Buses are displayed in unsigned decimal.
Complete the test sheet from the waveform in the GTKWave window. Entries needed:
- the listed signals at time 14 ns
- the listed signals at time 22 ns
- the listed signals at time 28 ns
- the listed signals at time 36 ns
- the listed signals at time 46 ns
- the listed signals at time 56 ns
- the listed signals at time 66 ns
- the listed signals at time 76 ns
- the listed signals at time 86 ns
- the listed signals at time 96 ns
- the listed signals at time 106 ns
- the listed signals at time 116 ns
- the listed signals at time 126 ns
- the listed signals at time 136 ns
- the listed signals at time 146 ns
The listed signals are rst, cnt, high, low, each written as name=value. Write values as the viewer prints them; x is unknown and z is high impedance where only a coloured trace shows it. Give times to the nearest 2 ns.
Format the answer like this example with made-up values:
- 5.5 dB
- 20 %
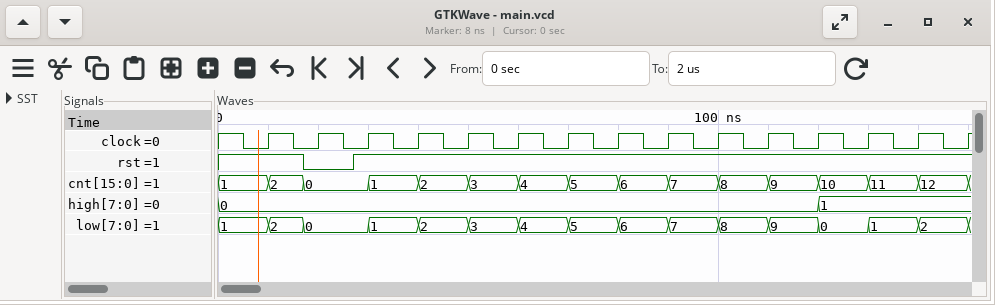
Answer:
- rst=1, cnt=2, high=0, low=2
- rst=0, cnt=0, high=0, low=0
- rst=1, cnt=0, high=0, low=0
- rst=1, cnt=1, high=0, low=1
- rst=1, cnt=2, high=0, low=2
- rst=1, cnt=3, high=0, low=3
- rst=1, cnt=4, high=0, low=4
- rst=1, cnt=5, high=0, low=5
- rst=1, cnt=6, high=0, low=6
- rst=1, cnt=7, high=0, low=7
- rst=1, cnt=8, high=0, low=8
- rst=1, cnt=9, high=0, low=9
- rst=1, cnt=10, high=1, low=0
- rst=1, cnt=11, high=1, low=1
- rst=1, cnt=12, high=1, low=2
